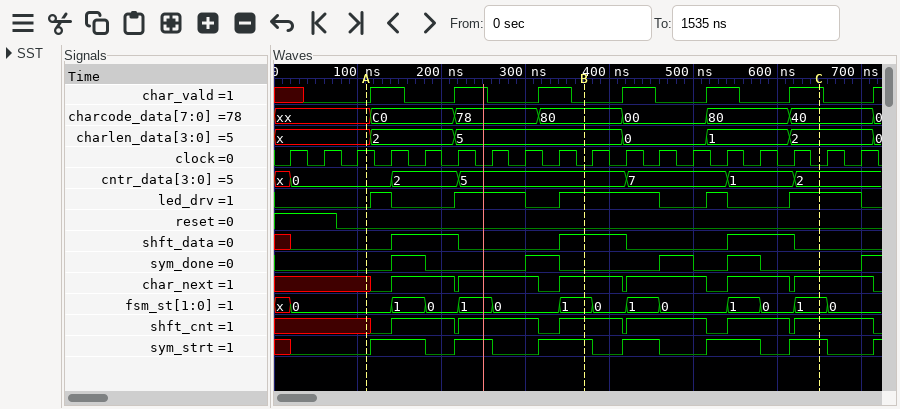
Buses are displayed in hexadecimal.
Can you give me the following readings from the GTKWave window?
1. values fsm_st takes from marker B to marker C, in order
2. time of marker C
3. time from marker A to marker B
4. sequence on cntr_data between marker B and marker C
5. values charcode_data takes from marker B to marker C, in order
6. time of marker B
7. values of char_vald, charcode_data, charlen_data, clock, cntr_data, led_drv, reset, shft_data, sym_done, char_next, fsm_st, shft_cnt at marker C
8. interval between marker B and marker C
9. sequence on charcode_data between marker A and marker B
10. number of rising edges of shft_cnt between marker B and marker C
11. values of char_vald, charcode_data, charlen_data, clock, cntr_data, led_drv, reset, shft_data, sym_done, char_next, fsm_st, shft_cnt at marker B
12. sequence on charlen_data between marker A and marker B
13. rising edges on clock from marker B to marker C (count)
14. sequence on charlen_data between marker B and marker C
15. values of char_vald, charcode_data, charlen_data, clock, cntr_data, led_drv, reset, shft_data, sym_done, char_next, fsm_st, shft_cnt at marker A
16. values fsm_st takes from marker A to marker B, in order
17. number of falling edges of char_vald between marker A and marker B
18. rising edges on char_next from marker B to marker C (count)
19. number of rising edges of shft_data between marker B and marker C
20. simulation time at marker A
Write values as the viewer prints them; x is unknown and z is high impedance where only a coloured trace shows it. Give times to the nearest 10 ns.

1, 0, 1, 0, 1, 0, 1
650 ns
260 ns
5, 7, 1, 2
80, 00, 80, 40
370 ns
char_vald=1, charcode_data=40, charlen_data=2, clock=0, cntr_data=2, led_drv=1, reset=0, shft_data=0, sym_done=0, char_next=1, fsm_st=1, shft_cnt=1
280 ns
xx, C0, 78, 80
3
char_vald=0, charcode_data=80, charlen_data=5, clock=0, cntr_data=5, led_drv=1, reset=0, shft_data=1, sym_done=0, char_next=1, fsm_st=1, shft_cnt=1
x, 2, 5
7
5, 0, 1, 2
char_vald=0, charcode_data=xx, charlen_data=x, clock=1, cntr_data=0, led_drv=0, reset=0, shft_data=0, sym_done=0, char_next=x, fsm_st=0, shft_cnt=x
0, 1, 0, 1, 0, 1
3
3
1
110 ns
